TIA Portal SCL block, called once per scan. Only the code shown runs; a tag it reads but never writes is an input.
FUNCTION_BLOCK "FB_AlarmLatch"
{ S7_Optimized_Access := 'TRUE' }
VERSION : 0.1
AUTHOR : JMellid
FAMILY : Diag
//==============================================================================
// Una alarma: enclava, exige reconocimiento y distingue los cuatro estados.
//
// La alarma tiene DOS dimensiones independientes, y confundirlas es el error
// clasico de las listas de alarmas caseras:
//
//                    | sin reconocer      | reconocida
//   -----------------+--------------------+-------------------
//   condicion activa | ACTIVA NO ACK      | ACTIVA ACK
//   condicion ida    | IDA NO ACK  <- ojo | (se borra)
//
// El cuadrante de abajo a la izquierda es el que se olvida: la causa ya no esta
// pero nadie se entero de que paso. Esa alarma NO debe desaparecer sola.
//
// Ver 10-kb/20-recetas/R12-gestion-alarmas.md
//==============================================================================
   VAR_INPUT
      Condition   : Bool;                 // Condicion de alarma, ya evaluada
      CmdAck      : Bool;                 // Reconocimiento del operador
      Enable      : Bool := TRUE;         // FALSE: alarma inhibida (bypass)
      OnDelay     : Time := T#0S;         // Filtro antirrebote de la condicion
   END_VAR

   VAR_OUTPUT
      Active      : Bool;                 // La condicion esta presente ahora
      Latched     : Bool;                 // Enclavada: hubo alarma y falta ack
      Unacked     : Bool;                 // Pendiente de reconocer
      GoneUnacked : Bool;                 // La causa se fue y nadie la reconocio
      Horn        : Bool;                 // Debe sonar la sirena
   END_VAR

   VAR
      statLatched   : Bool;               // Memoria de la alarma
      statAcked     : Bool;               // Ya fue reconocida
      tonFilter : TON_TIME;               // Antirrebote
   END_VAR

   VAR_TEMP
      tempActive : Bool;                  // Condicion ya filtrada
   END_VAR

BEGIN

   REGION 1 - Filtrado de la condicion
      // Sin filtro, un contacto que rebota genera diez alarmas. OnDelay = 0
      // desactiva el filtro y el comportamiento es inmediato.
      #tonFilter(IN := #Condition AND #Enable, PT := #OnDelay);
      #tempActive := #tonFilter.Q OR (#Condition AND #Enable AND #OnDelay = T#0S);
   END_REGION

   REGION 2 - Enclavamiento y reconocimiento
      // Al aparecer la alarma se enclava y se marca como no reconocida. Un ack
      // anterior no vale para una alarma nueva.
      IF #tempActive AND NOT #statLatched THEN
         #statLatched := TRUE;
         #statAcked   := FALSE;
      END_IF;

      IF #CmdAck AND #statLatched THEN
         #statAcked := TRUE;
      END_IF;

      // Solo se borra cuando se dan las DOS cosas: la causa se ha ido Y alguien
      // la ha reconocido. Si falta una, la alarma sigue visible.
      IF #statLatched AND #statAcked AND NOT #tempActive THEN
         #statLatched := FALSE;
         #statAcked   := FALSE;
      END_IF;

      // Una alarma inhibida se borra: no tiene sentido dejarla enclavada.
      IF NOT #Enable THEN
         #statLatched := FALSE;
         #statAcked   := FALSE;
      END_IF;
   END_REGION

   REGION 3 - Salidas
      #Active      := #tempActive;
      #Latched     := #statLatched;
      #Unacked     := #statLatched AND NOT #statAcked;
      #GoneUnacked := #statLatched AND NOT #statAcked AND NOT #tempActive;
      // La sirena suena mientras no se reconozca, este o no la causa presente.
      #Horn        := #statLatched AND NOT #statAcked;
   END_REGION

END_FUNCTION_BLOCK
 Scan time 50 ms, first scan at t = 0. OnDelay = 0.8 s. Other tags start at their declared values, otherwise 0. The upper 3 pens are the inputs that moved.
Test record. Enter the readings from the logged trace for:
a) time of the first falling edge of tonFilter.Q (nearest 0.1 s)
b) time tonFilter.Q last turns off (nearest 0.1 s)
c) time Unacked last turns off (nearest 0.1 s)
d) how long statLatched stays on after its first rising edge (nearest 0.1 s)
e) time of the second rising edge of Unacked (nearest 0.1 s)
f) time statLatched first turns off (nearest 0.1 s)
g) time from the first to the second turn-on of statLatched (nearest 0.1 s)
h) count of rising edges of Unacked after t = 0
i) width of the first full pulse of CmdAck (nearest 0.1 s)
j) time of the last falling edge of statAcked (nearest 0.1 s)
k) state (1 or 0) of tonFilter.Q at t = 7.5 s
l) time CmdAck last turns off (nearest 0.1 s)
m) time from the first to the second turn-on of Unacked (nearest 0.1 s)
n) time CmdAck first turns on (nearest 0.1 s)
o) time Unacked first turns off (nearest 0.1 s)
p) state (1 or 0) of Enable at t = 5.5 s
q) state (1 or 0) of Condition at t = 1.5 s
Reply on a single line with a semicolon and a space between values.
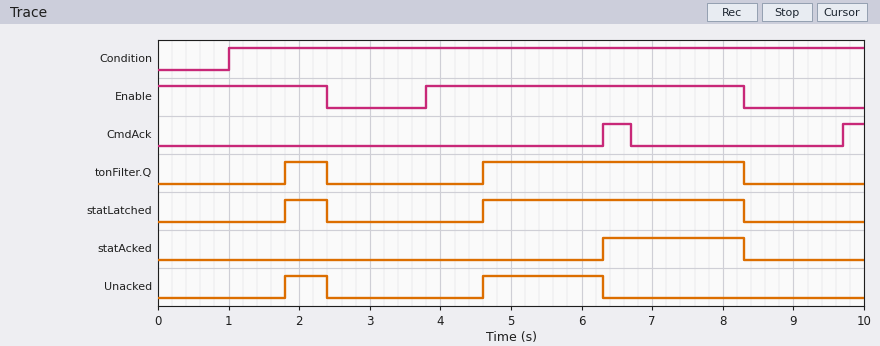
2.4 s; 8.3 s; 6.3 s; 0.6 s; 4.6 s; 2.4 s; 2.8 s; 2; 0.4 s; 8.3 s; 1; 6.7 s; 2.8 s; 6.3 s; 2.4 s; 1; 1
